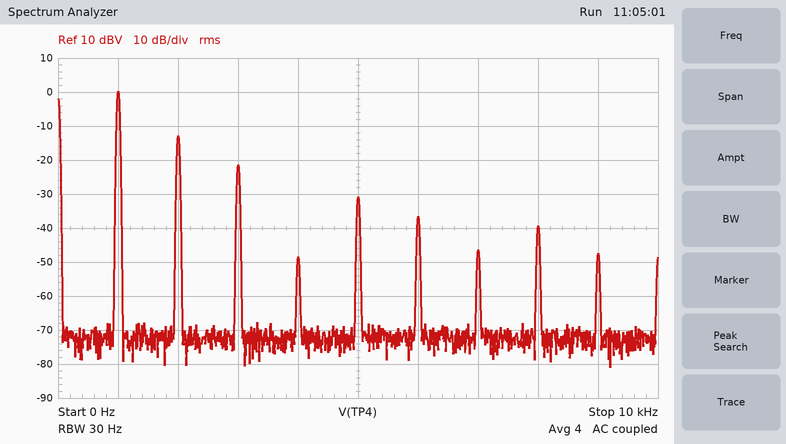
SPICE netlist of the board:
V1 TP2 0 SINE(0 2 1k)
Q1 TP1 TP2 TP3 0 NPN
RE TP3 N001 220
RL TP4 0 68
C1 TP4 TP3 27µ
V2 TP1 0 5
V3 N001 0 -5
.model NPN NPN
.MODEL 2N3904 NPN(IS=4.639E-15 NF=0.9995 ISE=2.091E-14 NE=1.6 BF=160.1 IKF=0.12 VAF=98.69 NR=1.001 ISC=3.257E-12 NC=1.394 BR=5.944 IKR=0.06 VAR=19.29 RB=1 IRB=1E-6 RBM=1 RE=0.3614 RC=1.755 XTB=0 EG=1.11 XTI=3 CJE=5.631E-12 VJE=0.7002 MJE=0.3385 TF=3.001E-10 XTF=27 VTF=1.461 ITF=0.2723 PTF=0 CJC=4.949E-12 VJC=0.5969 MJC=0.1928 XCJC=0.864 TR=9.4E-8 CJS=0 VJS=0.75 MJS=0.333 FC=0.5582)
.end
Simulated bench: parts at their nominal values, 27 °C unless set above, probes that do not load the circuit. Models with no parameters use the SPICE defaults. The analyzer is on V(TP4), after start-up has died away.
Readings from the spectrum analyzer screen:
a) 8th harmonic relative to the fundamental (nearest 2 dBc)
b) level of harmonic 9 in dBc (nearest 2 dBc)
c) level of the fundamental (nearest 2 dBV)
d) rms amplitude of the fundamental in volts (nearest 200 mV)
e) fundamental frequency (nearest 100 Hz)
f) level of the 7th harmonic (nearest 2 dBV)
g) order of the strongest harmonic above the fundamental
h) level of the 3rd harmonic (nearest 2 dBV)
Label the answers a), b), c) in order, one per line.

a) -40 dBc
b) -48 dBc
c) 0 dBV
d) 1.0 V
e) 1.0 kHz
f) -46 dBV
g) 2
h) -22 dBV
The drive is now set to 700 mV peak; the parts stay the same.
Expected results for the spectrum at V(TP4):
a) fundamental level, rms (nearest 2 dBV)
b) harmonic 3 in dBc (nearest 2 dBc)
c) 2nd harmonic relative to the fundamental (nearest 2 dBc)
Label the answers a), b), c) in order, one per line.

a) -6 dBV
b) -56 dBc
c) -44 dBc
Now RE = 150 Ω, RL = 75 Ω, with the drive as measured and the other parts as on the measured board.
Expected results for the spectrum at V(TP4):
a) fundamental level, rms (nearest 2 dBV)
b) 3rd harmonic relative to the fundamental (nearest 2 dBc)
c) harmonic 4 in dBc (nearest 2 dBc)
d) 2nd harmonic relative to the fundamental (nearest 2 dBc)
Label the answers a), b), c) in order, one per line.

a) 2 dBV
b) -24 dBc
c) -30 dBc
d) -20 dBc
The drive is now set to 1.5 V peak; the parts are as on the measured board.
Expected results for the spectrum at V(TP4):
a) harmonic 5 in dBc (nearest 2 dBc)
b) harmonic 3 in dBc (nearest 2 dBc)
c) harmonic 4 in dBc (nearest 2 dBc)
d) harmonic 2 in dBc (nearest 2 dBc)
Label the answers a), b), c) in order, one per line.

a) -56 dBc
b) -24 dBc
c) -32 dBc
d) -18 dBc
